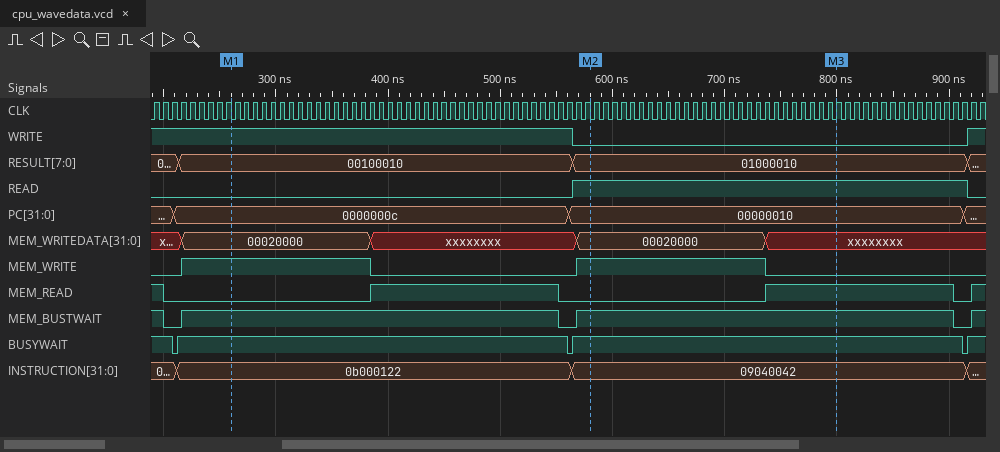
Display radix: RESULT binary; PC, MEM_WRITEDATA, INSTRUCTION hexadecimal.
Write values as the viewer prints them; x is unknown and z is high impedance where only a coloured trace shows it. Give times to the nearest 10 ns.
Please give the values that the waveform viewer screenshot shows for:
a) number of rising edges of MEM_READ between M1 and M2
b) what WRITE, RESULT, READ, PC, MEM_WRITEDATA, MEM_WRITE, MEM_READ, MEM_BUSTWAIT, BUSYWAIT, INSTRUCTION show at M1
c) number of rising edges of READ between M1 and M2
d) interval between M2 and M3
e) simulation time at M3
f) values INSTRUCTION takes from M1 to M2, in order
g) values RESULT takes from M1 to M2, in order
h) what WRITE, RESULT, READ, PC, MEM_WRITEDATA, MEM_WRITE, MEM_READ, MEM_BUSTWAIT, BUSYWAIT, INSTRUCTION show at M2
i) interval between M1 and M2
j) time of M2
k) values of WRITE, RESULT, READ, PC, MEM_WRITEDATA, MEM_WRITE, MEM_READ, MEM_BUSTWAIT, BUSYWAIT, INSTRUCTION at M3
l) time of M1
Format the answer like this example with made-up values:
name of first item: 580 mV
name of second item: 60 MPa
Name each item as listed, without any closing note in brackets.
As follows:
number of rising edges of MEM_READ between M1 and M2: 1
what WRITE, RESULT, READ, PC, MEM_WRITEDATA, MEM_WRITE, MEM_READ, MEM_BUSTWAIT, BUSYWAIT, INSTRUCTION show at M1: WRITE=1, RESULT=00100010, READ=0, PC=0000000c, MEM_WRITEDATA=00020000, MEM_WRITE=1, MEM_READ=0, MEM_BUSTWAIT=1, BUSYWAIT=1, INSTRUCTION=0b000122
number of rising edges of READ between M1 and M2: 1
interval between M2 and M3: 220 ns
simulation time at M3: 800 ns
values INSTRUCTION takes from M1 to M2, in order: 0b000122, 09040042
values RESULT takes from M1 to M2, in order: 00100010, 01000010
what WRITE, RESULT, READ, PC, MEM_WRITEDATA, MEM_WRITE, MEM_READ, MEM_BUSTWAIT, BUSYWAIT, INSTRUCTION show at M2: WRITE=0, RESULT=01000010, READ=1, PC=00000010, MEM_WRITEDATA=00020000, MEM_WRITE=1, MEM_READ=0, MEM_BUSTWAIT=1, BUSYWAIT=1, INSTRUCTION=09040042
interval between M1 and M2: 320 ns
time of M2: 580 ns
values of WRITE, RESULT, READ, PC, MEM_WRITEDATA, MEM_WRITE, MEM_READ, MEM_BUSTWAIT, BUSYWAIT, INSTRUCTION at M3: WRITE=0, RESULT=01000010, READ=1, PC=00000010, MEM_WRITEDATA=xxxxxxxx, MEM_WRITE=0, MEM_READ=1, MEM_BUSTWAIT=1, BUSYWAIT=1, INSTRUCTION=09040042
time of M1: 260 ns
